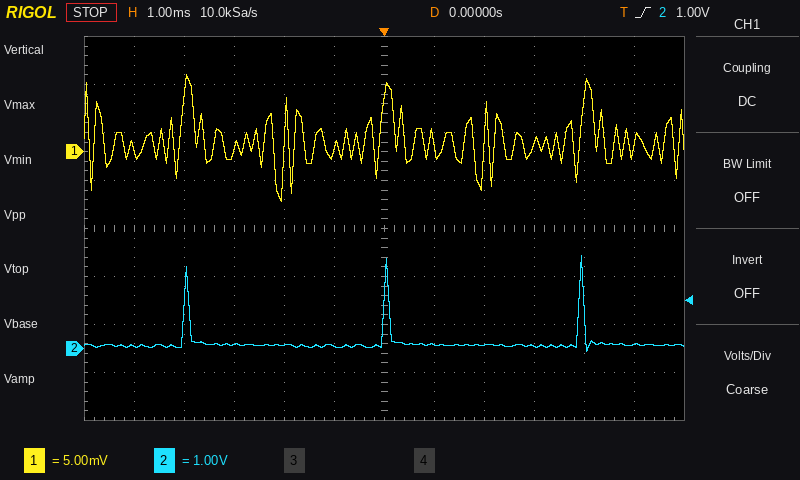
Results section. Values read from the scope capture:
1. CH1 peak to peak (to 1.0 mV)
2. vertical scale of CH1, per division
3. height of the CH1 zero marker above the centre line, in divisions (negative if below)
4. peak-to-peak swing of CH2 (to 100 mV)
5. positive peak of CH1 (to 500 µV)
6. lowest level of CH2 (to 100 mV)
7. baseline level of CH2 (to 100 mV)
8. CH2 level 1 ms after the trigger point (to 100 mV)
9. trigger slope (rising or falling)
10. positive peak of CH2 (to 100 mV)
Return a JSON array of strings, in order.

["13.0 mV", "5 mV", "+1.6 div", "2.0 V", "8.0 mV", "-100 mV", "100 mV", "100 mV", "rising", "1.9 V"]
